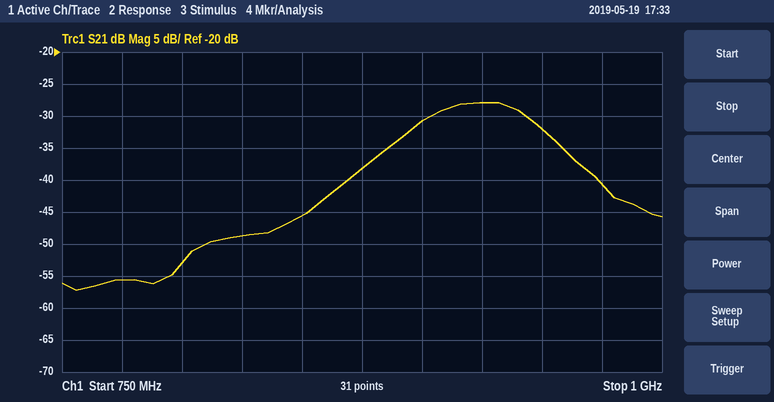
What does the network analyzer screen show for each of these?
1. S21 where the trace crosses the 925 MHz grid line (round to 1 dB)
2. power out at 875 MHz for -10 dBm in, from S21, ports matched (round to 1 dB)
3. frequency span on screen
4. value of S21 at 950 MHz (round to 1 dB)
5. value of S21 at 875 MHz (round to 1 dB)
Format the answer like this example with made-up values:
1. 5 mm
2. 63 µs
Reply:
1. -28 dB
2. -48 dBm
3. 250 MHz
4. -32 dB
5. -38 dB
